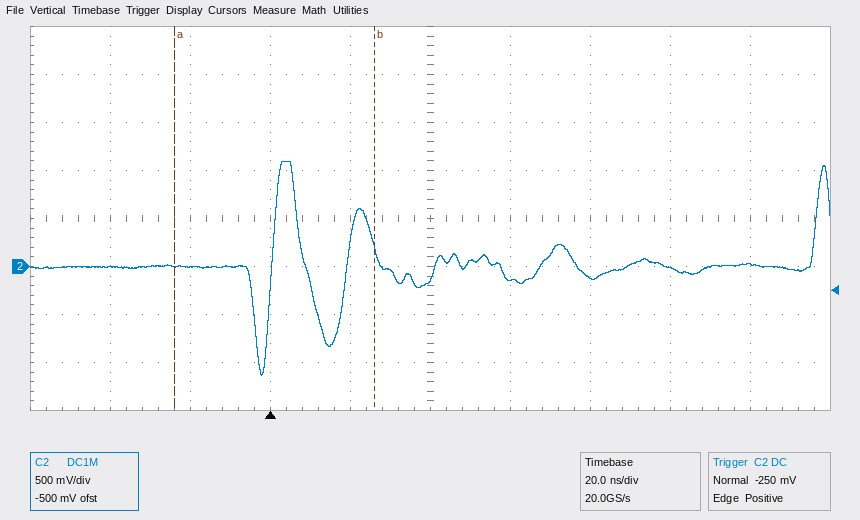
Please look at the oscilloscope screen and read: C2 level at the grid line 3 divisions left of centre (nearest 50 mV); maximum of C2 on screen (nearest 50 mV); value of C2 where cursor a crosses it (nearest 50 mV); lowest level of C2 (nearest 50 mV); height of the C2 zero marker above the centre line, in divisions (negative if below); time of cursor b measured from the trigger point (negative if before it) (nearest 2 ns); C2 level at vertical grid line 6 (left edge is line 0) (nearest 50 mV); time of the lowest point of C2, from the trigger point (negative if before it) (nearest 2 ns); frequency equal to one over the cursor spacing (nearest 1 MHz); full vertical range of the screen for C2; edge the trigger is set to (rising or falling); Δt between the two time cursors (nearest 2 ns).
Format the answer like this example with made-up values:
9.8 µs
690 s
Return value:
0 mV
1.10 V
0 mV
-1.15 V
-1.0 div
+26 ns
-150 mV
-2 ns
20 MHz
4 V
rising
50 ns
